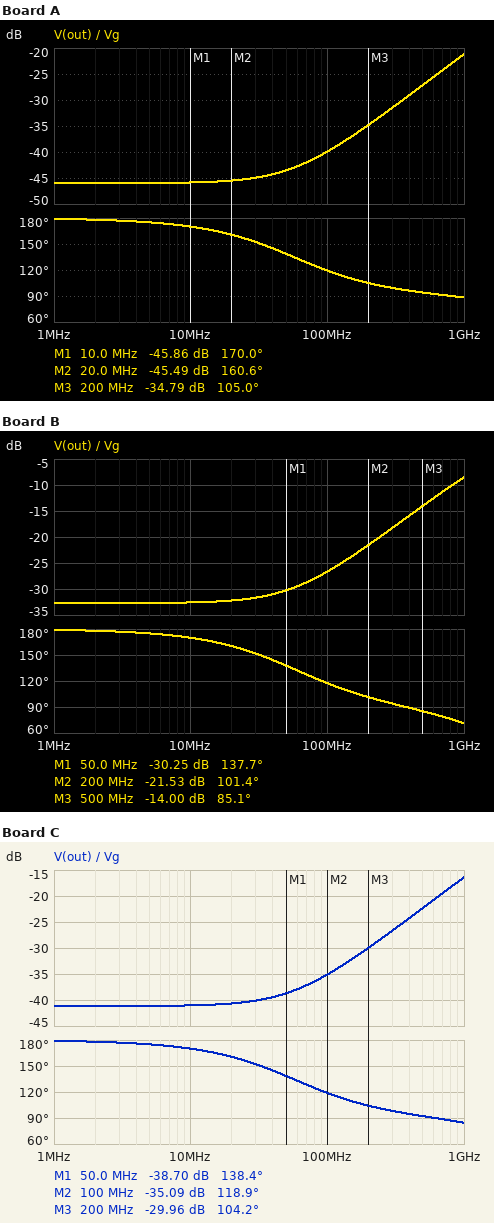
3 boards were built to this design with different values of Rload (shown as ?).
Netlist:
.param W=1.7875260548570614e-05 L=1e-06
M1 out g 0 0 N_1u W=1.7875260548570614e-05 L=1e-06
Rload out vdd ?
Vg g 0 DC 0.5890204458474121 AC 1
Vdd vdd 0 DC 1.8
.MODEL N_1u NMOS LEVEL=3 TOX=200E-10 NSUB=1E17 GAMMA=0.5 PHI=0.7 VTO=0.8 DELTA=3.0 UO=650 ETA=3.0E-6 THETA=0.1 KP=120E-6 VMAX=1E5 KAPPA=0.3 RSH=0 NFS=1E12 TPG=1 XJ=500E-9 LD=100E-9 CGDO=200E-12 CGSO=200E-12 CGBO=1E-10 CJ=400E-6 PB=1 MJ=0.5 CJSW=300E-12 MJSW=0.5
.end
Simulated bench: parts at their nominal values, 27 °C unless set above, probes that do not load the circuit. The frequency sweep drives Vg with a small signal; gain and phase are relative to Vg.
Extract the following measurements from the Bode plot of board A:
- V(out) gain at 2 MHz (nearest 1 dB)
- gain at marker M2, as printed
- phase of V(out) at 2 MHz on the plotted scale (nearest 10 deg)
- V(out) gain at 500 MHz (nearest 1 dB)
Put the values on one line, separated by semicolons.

-46 dB; -45.49 dB; 180 deg; -27 dB
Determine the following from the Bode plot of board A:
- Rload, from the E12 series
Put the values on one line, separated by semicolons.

3.9 kΩ
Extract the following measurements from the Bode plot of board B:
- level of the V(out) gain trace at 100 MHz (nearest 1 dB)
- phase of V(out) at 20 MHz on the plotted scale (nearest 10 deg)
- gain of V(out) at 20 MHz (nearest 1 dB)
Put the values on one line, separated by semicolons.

-27 dB; 160 deg; -32 dB
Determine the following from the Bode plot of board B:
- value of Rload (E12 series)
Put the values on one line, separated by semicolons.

18 kΩ
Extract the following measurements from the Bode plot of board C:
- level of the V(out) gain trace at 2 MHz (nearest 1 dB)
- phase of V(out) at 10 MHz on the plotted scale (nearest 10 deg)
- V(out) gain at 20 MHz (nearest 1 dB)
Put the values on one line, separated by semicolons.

-41 dB; 170 deg; -41 dB
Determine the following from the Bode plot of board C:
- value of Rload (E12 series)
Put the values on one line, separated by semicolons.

6.8 kΩ
